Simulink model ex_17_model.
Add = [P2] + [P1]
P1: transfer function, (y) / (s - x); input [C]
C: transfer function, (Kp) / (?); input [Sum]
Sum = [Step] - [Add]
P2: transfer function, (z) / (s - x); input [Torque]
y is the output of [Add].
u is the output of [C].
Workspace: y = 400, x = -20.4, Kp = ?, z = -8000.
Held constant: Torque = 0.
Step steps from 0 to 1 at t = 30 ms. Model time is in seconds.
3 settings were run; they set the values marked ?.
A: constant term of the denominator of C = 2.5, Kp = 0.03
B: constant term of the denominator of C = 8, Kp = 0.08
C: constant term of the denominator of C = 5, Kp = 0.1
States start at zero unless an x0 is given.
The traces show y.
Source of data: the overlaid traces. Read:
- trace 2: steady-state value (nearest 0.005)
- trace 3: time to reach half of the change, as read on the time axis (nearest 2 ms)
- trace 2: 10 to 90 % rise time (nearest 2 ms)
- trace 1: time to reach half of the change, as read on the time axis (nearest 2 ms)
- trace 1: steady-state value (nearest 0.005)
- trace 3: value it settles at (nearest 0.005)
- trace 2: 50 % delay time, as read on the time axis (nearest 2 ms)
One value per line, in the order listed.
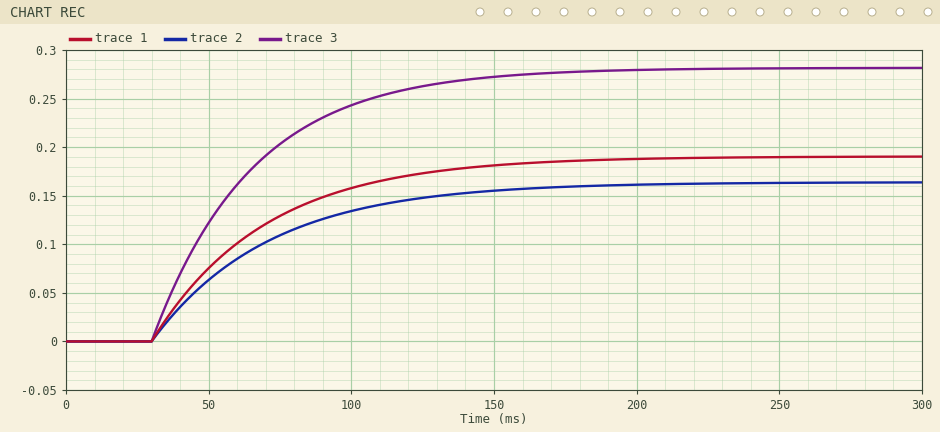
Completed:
0.165
54 ms
90 ms
58 ms
0.190
0.280
58 ms
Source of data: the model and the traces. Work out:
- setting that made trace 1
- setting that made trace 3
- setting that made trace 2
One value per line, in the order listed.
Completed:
A
C
B
